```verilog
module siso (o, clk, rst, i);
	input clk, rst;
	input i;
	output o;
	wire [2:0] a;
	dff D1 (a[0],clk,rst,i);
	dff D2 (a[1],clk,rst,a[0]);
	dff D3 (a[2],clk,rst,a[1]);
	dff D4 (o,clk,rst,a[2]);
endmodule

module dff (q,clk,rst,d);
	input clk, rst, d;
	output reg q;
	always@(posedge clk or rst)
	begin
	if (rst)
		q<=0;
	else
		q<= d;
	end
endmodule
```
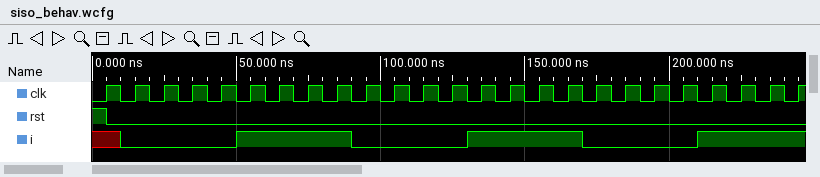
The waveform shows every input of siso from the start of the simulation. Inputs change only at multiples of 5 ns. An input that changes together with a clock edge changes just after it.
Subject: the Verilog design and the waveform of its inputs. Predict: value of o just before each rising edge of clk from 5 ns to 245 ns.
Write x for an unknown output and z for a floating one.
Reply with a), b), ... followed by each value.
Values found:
a) 0 0 0 0 x 0 0 0 0 1 1 1 1 0 0 0 0 1 1 1 1 0 0 0 0
